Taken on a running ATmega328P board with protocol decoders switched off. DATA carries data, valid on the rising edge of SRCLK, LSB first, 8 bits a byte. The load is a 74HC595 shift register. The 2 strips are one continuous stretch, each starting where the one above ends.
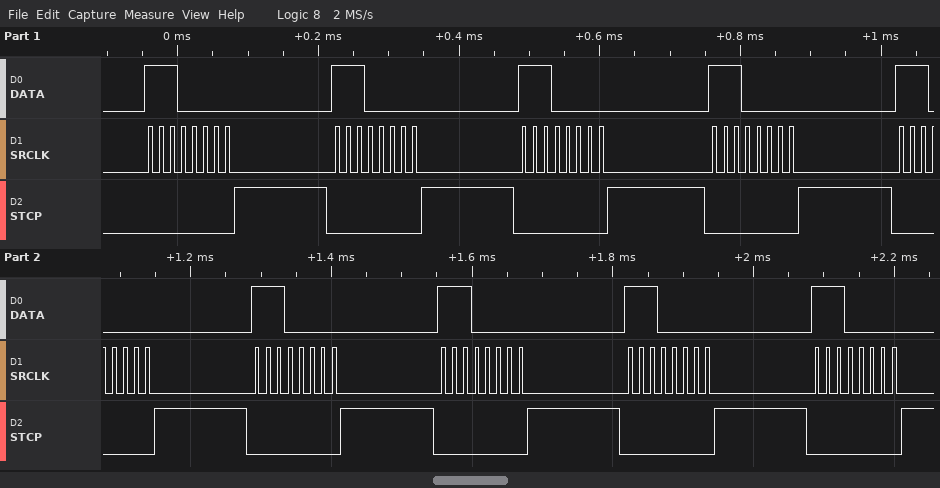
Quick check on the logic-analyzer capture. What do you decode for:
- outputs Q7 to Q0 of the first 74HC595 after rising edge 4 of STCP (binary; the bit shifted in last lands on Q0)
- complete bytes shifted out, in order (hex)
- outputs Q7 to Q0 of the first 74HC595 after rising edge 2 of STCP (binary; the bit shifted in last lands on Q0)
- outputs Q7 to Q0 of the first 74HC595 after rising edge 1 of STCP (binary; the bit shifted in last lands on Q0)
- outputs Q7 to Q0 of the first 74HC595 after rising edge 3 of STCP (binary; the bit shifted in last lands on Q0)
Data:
11100000
0x07 0x07 0x07 0x07 0x07 0x07 0x07 0x07 0x07
11100000
11100000
11100000
